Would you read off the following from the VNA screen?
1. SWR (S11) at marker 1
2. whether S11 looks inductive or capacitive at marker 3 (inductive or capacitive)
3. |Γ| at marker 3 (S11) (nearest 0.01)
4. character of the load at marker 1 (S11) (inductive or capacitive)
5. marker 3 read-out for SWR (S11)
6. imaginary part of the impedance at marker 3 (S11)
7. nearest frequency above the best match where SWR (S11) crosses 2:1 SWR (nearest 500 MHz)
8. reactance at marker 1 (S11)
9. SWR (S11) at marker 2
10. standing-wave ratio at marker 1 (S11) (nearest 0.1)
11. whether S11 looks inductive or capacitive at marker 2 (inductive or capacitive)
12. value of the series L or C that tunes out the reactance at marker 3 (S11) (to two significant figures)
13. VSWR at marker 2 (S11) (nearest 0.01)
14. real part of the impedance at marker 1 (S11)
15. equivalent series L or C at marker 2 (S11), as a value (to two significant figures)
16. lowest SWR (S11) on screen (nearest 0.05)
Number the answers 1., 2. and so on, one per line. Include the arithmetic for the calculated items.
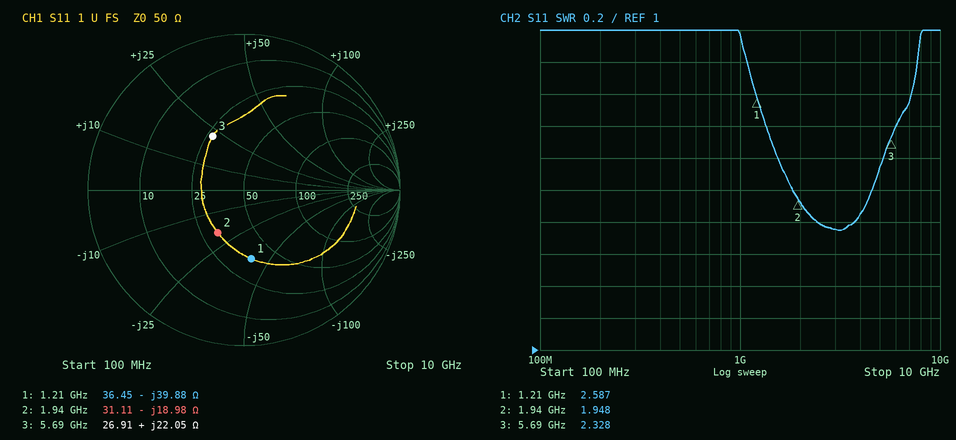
1. 2.587
2. inductive
3. 0.40
4. capacitive
5. 2.328
6. +22.05 Ω
7. 4.5 GHz
8. -39.88 Ω
9. 1.948
10. 2.6
11. capacitive
12. C = 1/(2π × 5.69 GHz × 22.05 Ω) ≈ 1.3 pF
13. 1.95
14. 36.45 Ω
15. C = 1/(2π × 1.94 GHz × 18.98 Ω) ≈ 4.3 pF
16. 1.75
